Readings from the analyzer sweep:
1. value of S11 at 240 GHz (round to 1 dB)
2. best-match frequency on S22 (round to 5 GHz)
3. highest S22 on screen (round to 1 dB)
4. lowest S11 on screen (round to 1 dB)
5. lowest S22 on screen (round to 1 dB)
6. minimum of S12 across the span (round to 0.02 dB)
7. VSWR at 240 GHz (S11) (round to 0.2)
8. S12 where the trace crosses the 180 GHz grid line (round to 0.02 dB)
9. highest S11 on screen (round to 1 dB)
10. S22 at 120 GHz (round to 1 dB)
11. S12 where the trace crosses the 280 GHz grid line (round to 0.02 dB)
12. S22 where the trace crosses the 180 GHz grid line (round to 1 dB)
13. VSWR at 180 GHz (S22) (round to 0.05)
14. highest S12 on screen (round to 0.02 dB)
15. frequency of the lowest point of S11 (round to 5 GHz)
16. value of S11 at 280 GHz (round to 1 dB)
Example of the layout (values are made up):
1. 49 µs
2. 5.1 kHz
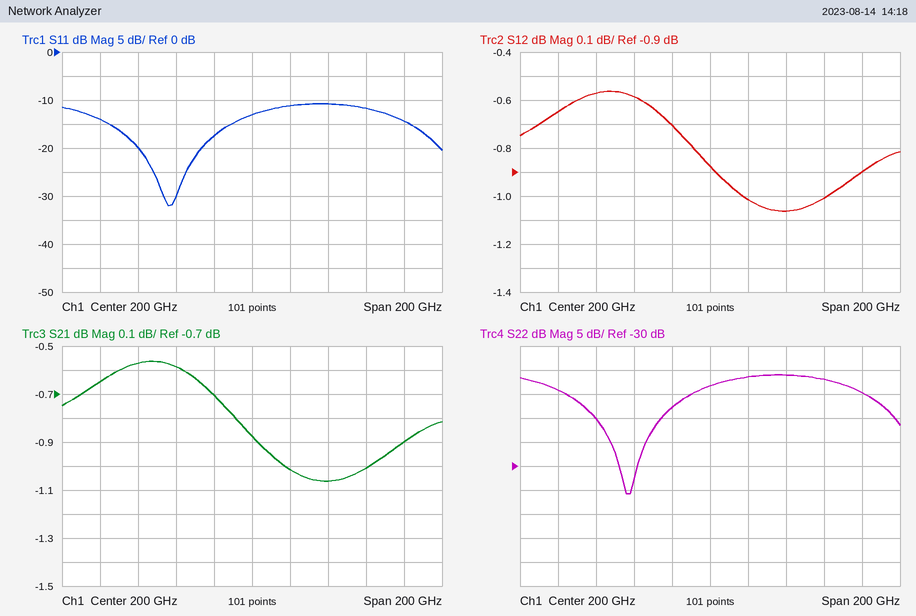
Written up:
1. -11 dB
2. 155 GHz
3. -11 dB
4. -32 dB
5. -36 dB
6. -1.06 dB
7. 1.8
8. -0.70 dB
9. -11 dB
10. -14 dB
11. -0.90 dB
12. -18 dB
13. 1.30
14. -0.56 dB
15. 155 GHz
16. -14 dB
